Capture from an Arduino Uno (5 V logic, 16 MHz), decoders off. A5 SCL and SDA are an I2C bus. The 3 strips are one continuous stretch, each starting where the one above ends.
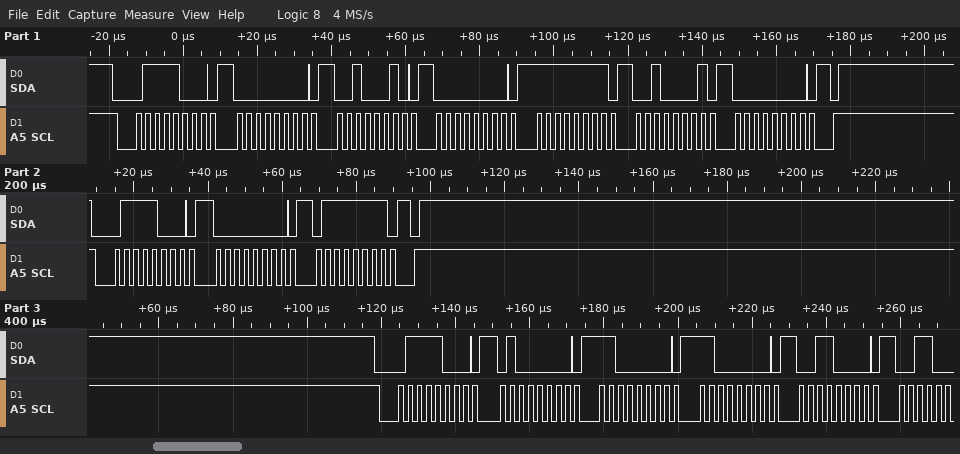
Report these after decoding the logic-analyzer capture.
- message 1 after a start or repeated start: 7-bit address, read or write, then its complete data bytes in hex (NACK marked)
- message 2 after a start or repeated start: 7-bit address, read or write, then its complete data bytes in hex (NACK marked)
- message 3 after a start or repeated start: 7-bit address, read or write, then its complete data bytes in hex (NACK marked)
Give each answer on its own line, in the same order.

0x3C write: 00 22 00 FF 21 00
0x3C write: 00 7F
0x3C write: 40 C0 C0 30
